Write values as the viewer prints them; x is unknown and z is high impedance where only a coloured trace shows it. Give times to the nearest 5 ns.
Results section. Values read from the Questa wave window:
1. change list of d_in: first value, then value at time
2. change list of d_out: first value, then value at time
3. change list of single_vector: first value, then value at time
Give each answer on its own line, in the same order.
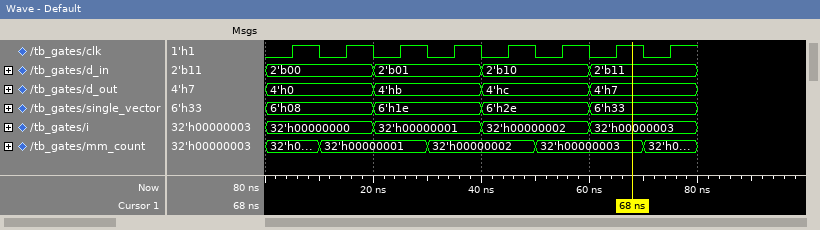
2'b00, 2'b01 at 20 ns, 2'b10 at 40 ns, 2'b11 at 60 ns
4'h0, 4'hb at 20 ns, 4'hc at 40 ns, 4'h7 at 60 ns
6'h08, 6'h1e at 20 ns, 6'h2e at 40 ns, 6'h33 at 60 ns
